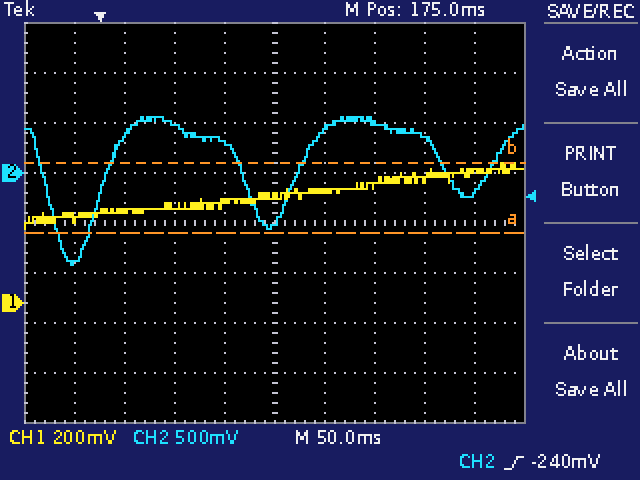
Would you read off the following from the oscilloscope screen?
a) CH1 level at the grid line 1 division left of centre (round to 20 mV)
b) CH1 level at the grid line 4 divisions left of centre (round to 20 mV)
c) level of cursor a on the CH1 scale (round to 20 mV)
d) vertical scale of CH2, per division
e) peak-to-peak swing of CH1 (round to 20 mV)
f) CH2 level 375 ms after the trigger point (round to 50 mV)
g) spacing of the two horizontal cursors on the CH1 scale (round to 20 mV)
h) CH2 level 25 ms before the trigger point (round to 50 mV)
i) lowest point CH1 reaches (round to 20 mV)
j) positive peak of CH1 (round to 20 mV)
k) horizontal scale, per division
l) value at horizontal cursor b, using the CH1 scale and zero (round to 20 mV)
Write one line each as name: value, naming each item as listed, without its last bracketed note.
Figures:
CH1 level at the grid line 1 division left of centre: 400 mV
CH1 level at the grid line 4 divisions left of centre: 340 mV
level of cursor a on the CH1 scale: 280 mV
vertical scale of CH2, per division: 500 mV
peak-to-peak swing of CH1: 260 mV
CH2 level 375 ms after the trigger point: -200 mV
spacing of the two horizontal cursors on the CH1 scale: 280 mV
CH2 level 25 ms before the trigger point: -900 mV
lowest point CH1 reaches: 300 mV
positive peak of CH1: 560 mV
horizontal scale, per division: 50 ms
value at horizontal cursor b, using the CH1 scale and zero: 560 mV
